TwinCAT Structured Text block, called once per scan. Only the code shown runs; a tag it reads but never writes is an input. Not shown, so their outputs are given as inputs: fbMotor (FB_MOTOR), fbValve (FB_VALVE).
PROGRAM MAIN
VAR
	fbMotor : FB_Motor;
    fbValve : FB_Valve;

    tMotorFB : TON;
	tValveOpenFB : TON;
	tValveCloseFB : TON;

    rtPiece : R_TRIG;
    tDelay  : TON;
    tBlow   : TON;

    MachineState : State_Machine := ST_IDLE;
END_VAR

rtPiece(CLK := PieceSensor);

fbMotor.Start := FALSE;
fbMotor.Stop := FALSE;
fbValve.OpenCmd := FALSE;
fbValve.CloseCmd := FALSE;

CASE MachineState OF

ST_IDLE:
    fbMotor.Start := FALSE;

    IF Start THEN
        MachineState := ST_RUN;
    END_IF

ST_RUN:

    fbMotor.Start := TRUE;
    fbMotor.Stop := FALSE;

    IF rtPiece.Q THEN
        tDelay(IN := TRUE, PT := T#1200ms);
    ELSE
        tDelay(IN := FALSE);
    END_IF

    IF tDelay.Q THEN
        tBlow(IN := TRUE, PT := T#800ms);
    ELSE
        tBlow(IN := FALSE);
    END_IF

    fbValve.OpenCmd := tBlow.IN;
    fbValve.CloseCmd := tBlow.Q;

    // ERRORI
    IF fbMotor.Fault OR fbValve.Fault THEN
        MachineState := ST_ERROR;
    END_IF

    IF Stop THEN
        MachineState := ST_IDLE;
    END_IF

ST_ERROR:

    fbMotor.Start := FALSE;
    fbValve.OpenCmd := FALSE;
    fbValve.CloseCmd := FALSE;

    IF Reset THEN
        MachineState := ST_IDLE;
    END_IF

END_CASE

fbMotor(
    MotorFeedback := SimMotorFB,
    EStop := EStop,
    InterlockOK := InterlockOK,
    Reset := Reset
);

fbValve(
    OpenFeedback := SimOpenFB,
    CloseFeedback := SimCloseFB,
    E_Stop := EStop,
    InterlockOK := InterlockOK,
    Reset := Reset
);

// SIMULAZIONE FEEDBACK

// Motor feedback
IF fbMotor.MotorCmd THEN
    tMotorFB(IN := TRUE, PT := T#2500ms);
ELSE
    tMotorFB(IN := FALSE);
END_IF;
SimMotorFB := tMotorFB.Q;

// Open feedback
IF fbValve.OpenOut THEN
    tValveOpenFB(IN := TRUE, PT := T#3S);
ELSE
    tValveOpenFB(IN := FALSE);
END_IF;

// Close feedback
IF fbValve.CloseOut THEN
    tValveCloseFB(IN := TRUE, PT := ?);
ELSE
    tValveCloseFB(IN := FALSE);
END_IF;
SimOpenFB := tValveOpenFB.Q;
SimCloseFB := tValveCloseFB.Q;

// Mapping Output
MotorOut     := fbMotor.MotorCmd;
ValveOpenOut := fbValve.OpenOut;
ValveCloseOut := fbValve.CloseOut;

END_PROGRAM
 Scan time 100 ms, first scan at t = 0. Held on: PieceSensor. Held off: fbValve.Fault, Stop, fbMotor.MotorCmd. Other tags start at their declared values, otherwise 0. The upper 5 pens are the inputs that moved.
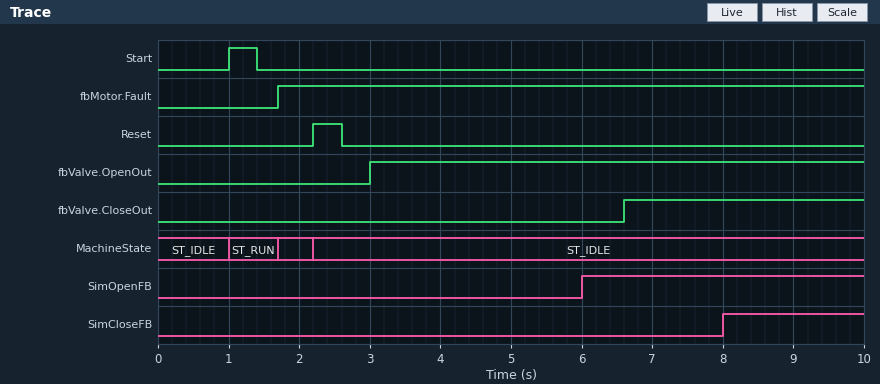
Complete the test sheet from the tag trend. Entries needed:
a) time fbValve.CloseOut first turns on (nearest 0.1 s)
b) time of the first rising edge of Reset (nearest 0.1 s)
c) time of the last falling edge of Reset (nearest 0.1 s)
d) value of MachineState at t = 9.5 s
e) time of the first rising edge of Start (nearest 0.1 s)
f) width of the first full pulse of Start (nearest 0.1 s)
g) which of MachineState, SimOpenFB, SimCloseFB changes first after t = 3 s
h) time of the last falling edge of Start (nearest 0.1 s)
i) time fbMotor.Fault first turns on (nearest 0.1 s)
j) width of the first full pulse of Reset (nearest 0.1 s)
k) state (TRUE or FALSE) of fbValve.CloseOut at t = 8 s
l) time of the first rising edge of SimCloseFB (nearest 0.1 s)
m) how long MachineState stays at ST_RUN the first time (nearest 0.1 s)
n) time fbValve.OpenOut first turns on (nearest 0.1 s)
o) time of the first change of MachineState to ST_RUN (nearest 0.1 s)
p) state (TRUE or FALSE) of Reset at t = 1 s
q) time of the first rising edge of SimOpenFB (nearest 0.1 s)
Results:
6.6 s
2.2 s
2.6 s
ST_IDLE
1.0 s
0.4 s
SimOpenFB
1.4 s
1.7 s
0.4 s
TRUE
8.0 s
0.7 s
3.0 s
1.0 s
FALSE
6.0 s
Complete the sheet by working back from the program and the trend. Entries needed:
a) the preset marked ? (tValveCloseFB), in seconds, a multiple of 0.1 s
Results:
1.4 s
